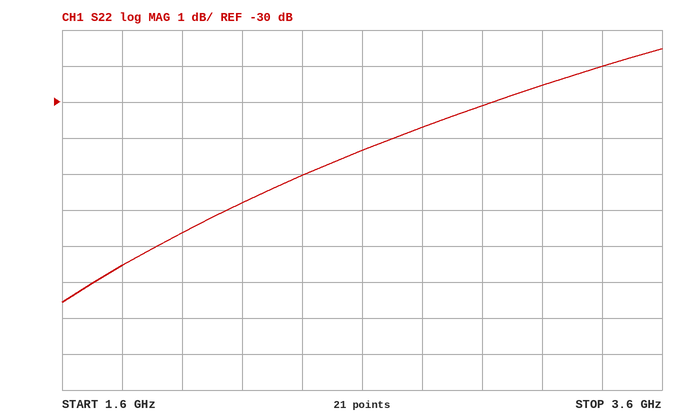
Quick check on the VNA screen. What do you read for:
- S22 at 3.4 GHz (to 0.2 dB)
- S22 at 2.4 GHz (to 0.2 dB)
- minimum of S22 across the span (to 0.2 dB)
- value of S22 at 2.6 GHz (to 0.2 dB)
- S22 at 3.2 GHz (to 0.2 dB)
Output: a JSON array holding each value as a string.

["-29.0 dB", "-32.0 dB", "-35.6 dB", "-31.4 dB", "-29.6 dB"]
